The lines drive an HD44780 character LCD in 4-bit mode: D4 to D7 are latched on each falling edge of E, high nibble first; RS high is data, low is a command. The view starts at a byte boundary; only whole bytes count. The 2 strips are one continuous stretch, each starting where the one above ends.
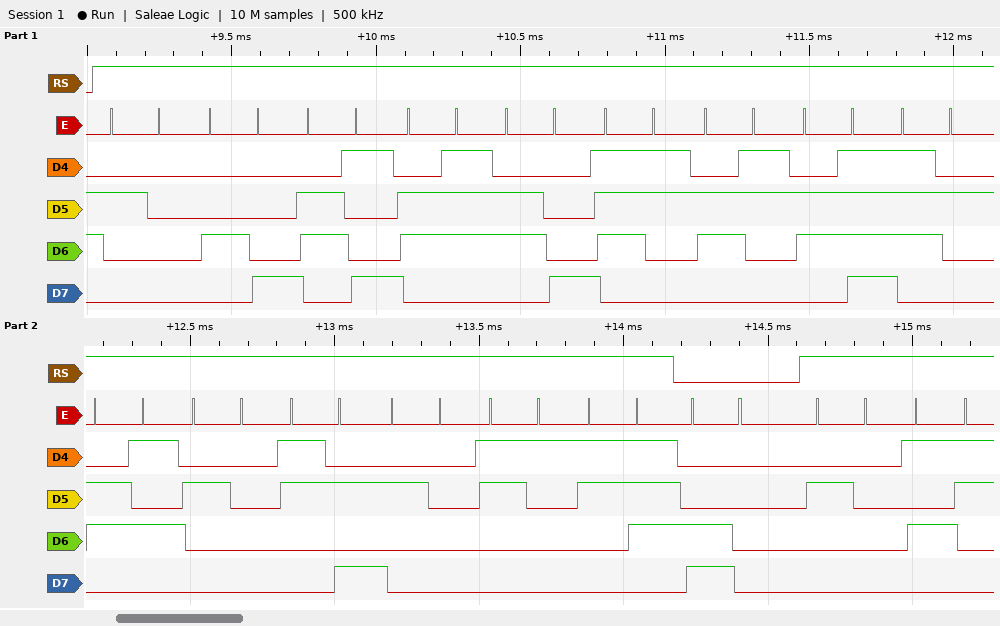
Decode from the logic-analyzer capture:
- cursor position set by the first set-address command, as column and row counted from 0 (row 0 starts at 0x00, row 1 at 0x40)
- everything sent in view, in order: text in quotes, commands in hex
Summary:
column 0, row 1
" Highscore : 17" 0xC0 " S"
